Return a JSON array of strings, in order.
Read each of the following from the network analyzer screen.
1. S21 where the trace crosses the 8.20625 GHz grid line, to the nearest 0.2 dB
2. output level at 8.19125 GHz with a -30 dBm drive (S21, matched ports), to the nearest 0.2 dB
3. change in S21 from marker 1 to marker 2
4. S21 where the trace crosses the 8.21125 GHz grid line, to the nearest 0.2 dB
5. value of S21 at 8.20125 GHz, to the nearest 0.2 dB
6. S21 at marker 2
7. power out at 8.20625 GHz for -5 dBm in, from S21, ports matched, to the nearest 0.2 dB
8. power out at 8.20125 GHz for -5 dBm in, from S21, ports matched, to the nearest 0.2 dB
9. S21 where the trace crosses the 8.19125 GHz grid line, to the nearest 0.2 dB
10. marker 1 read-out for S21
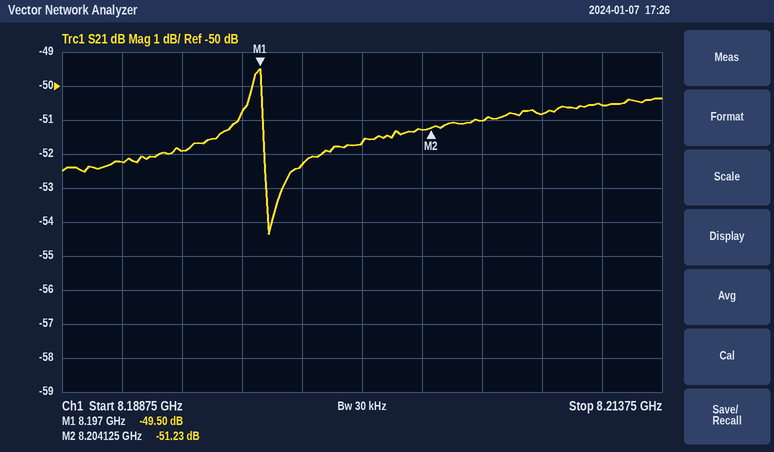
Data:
["-51.0 dB", "-82.2 dBm", "-1.73 dB", "-50.6 dB", "-51.6 dB", "-51.23 dB", "-56.0 dBm", "-56.6 dBm", "-52.2 dB", "-49.50 dB"]
